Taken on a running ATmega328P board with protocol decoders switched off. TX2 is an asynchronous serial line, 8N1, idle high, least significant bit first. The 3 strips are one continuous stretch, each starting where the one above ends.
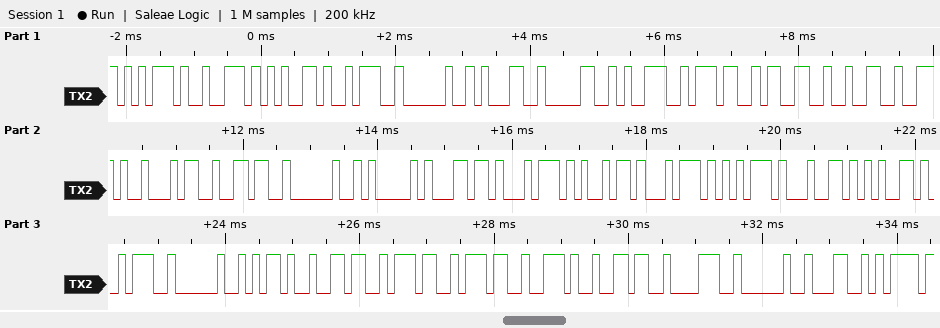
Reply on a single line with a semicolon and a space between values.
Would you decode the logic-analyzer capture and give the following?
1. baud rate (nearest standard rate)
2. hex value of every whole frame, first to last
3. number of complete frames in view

9600 baud; 75 72 65 3A 20 31 30 39 37 33 32 2E 34 36 20 41 6C 74 69 74 75 64 65 3A 20 2D 36 37 37 2E 36 38 20 4C; 34
